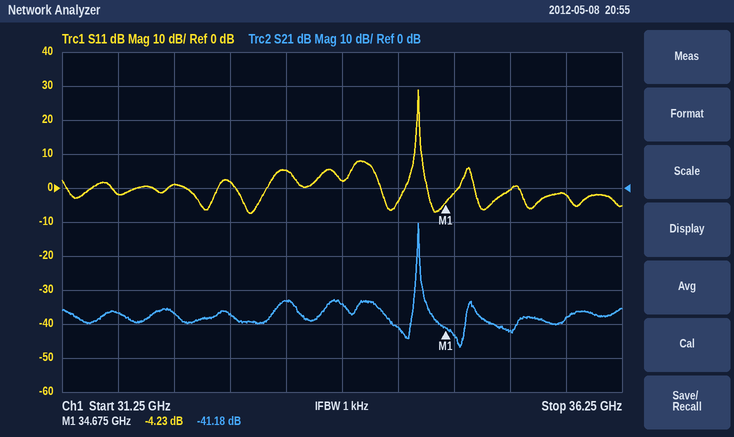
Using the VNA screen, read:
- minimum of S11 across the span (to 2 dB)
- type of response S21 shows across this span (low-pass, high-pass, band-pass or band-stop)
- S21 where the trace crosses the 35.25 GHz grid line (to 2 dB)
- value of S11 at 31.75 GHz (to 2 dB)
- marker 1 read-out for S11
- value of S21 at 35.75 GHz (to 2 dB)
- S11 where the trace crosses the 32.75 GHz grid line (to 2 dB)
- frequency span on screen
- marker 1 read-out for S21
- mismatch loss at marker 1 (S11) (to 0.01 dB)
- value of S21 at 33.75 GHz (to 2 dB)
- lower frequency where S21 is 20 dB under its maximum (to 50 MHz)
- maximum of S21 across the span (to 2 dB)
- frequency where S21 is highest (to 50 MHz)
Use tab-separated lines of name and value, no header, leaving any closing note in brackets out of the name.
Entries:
minimum of S11 across the span	-8 dB
type of response S21 shows across this span	band-pass
S21 where the trace crosses the 35.25 GHz grid line	-42 dB
value of S11 at 31.75 GHz	-2 dB
marker 1 read-out for S11	-4.23 dB
value of S21 at 35.75 GHz	-38 dB
S11 where the trace crosses the 32.75 GHz grid line	2 dB
frequency span on screen	5 GHz
marker 1 read-out for S21	-41.18 dB
mismatch loss at marker 1 (S11)	2.06 dB
value of S21 at 33.75 GHz	-34 dB
lower frequency where S21 is 20 dB under its maximum	34.40 GHz
maximum of S21 across the span	-10 dB
frequency where S21 is highest	34.45 GHz
